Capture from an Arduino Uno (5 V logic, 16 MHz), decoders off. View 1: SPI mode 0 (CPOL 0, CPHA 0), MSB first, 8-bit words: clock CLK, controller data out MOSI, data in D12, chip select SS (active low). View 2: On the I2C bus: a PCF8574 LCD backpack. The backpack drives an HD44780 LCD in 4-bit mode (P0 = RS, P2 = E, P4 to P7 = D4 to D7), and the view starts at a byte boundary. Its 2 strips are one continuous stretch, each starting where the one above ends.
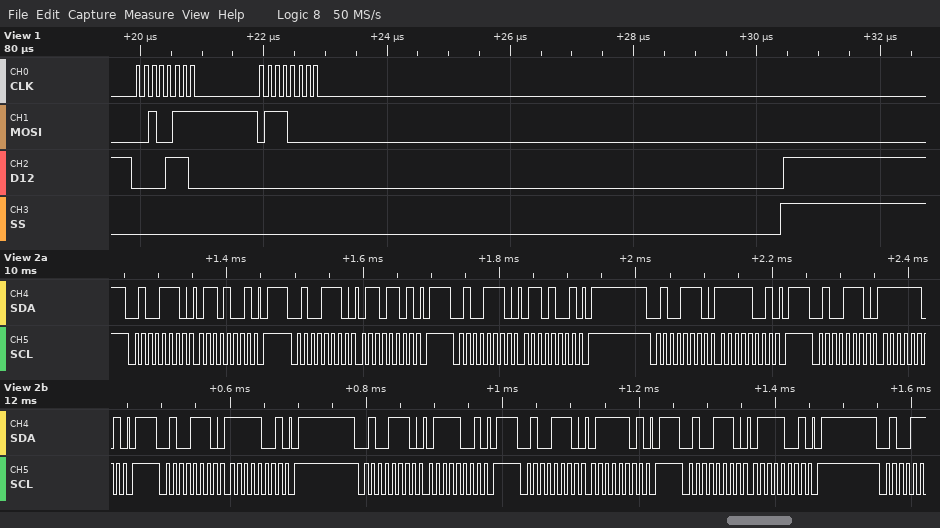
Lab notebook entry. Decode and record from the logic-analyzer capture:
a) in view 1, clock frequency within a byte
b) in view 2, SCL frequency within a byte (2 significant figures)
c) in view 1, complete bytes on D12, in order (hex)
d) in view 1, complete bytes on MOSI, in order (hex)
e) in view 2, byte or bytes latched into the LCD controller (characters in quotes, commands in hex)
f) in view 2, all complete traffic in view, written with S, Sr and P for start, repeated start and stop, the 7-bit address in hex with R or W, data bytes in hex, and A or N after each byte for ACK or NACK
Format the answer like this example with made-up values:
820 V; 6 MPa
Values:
8 MHz; 100 kHz; 0E 00; 27 70; 'o'; S 27W A 69 A P S 27W A 6D A P S 27W A 69 A P S 27W A F9 A P S 27W A FD A P S 27W A F9 A P S 27W A 79 A P S 27W A 7D A P S 27W A 79 A P
